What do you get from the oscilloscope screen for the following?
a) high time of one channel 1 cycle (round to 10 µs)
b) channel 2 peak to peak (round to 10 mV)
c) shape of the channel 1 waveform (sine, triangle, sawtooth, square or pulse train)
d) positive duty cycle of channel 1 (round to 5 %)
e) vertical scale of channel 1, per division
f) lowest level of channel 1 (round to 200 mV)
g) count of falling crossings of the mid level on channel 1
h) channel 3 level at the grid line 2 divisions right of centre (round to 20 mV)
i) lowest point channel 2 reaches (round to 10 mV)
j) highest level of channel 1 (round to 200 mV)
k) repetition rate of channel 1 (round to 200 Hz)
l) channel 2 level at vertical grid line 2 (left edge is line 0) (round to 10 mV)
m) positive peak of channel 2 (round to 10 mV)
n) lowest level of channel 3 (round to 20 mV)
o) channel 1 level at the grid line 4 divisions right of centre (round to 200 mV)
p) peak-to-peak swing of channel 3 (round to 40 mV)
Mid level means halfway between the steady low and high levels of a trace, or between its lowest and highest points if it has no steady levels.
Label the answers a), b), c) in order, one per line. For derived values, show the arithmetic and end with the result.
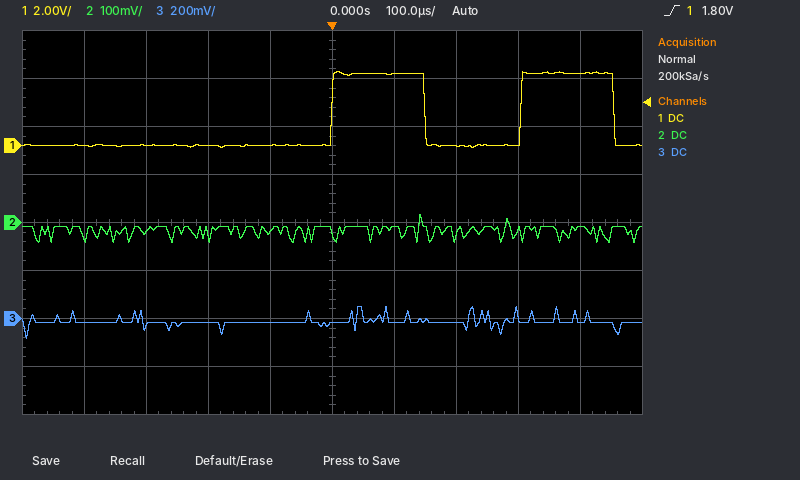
a) 150 µs
b) 20 mV − (-40 mV) = 60 mV
c) square
d) 50 %
e) 2 V
f) 0.0 V
g) 2
h) -20 mV
i) -40 mV
j) 3.0 V
k) 3.2 kHz
l) -20 mV
m) 20 mV
n) -80 mV
o) 3.0 V
p) 120 mV
